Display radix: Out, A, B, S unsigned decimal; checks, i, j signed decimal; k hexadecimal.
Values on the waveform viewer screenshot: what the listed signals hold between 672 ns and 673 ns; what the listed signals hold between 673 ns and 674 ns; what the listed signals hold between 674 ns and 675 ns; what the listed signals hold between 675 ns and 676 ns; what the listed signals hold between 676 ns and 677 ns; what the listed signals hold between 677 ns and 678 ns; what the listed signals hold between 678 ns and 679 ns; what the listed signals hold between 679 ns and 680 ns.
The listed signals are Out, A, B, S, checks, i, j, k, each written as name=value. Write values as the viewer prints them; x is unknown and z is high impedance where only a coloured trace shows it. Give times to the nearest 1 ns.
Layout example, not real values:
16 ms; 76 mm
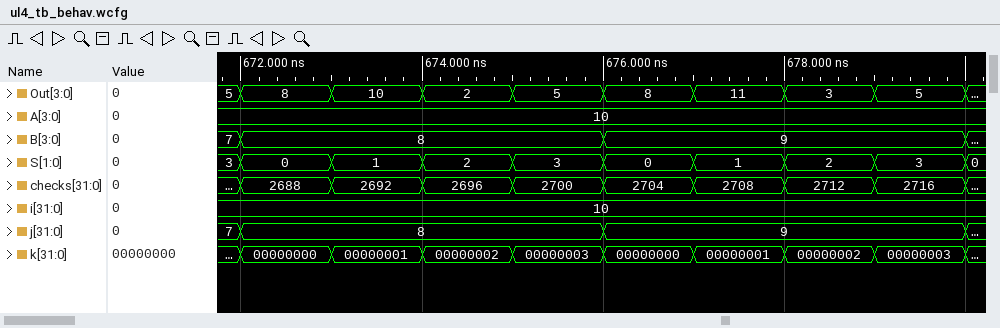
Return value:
Out=8, A=10, B=8, S=0, checks=2688, i=10, j=8, k=00000000; Out=10, A=10, B=8, S=1, checks=2692, i=10, j=8, k=00000001; Out=2, A=10, B=8, S=2, checks=2696, i=10, j=8, k=00000002; Out=5, A=10, B=8, S=3, checks=2700, i=10, j=8, k=00000003; Out=8, A=10, B=9, S=0, checks=2704, i=10, j=9, k=00000000; Out=11, A=10, B=9, S=1, checks=2708, i=10, j=9, k=00000001; Out=3, A=10, B=9, S=2, checks=2712, i=10, j=9, k=00000002; Out=5, A=10, B=9, S=3, checks=2716, i=10, j=9, k=00000003
